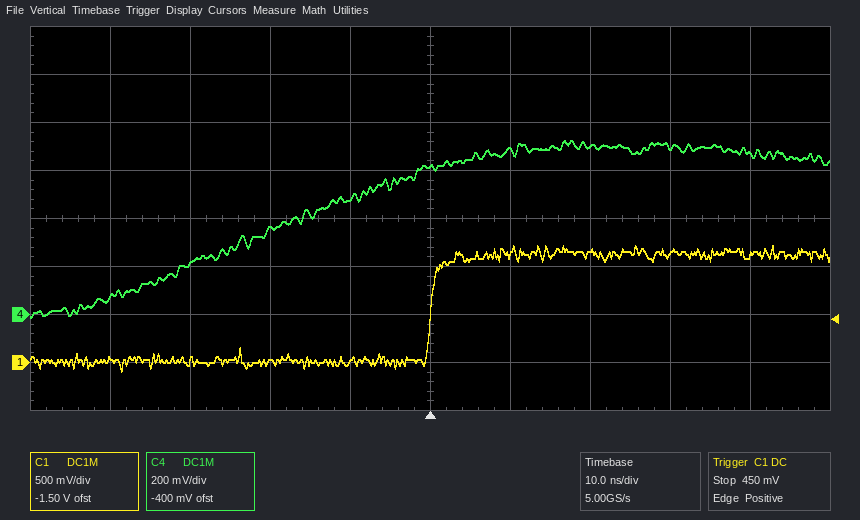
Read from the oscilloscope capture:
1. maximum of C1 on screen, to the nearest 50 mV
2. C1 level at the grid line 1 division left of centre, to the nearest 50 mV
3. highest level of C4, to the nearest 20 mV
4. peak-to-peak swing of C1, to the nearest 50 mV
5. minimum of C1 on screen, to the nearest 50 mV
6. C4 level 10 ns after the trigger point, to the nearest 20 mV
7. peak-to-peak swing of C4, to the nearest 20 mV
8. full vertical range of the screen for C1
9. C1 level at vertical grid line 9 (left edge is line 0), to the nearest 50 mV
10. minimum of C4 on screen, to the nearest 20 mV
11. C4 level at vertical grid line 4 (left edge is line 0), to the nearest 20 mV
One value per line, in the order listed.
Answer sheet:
1.20 V
0 mV
720 mV
1.30 V
-100 mV
680 mV
740 mV
4 V
1.10 V
-20 mV
480 mV
